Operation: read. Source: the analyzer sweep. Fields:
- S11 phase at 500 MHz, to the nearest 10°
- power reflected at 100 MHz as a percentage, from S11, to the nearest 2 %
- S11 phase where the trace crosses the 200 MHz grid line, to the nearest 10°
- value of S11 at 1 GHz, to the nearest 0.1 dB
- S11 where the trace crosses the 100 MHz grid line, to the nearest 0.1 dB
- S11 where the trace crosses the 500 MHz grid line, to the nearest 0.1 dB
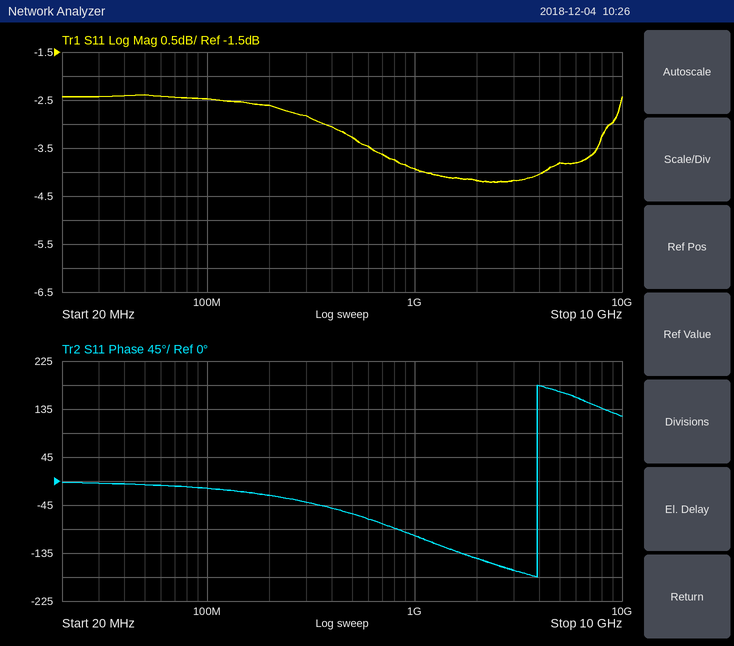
-60°
56 %
-30°
-3.9 dB
-2.5 dB
-3.3 dB
